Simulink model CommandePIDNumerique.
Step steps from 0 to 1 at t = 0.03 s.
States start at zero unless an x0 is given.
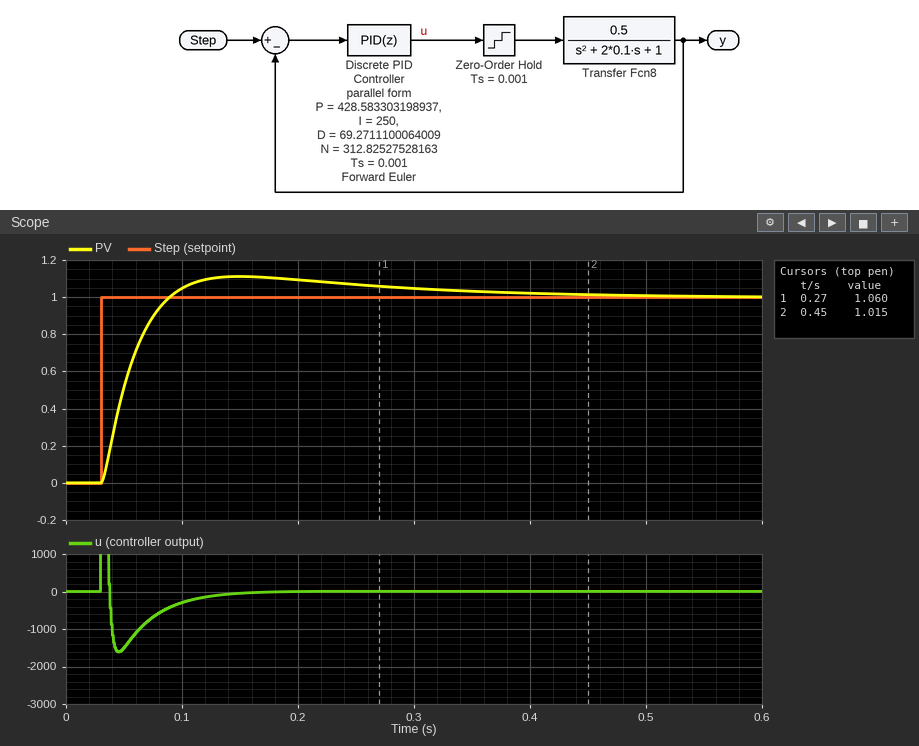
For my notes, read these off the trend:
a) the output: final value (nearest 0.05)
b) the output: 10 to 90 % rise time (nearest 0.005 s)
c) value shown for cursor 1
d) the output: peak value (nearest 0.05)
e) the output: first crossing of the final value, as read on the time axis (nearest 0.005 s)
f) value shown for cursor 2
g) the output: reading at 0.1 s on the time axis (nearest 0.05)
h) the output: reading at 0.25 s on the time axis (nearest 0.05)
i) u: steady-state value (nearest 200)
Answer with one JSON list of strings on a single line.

["1.00", "0.040 s", "1.060", "1.10", "0.090 s", "1.015", "1.05", "1.05", "0"]
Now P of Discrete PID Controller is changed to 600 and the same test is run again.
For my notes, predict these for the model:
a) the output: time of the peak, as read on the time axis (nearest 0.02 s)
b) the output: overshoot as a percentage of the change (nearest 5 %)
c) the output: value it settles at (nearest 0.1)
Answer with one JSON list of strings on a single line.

["0.14 s", "15 %", "1.0"]
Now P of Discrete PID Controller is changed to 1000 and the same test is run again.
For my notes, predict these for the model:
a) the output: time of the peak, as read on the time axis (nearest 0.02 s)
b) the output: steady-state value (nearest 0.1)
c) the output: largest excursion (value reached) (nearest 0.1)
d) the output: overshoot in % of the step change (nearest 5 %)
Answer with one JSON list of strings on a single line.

["0.12 s", "1.0", "1.2", "20 %"]
